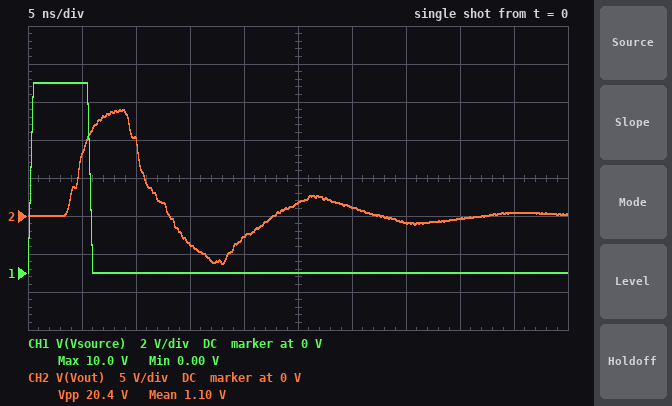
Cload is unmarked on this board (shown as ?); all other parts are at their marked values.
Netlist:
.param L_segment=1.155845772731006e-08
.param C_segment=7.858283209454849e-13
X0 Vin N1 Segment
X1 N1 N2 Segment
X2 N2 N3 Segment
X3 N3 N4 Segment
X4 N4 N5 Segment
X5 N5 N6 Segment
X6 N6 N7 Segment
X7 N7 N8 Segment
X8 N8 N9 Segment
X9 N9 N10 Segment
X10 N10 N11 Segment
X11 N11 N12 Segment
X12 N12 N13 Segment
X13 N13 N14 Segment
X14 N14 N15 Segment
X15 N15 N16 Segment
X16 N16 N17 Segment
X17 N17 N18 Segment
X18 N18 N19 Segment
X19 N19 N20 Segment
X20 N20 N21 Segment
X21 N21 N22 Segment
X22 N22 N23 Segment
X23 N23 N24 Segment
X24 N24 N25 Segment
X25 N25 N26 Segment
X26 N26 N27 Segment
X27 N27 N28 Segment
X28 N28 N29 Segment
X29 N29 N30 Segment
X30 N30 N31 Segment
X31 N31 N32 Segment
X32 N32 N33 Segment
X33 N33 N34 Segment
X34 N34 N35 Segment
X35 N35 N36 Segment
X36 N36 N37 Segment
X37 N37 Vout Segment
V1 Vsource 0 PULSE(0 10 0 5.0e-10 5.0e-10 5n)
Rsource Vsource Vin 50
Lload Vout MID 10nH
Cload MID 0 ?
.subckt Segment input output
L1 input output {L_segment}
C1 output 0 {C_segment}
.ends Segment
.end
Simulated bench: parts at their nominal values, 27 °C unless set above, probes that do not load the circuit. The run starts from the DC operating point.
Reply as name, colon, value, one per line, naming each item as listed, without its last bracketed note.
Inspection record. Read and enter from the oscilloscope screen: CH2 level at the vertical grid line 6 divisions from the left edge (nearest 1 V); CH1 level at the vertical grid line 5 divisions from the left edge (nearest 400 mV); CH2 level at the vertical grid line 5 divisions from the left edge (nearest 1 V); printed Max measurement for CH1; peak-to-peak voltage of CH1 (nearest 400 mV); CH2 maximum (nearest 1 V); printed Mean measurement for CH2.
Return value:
CH2 level at the vertical grid line 6 divisions from the left edge: 1 V
CH1 level at the vertical grid line 5 divisions from the left edge: 0 V
CH2 level at the vertical grid line 5 divisions from the left edge: 2 V
printed Max measurement for CH1: 10.0 V
peak-to-peak voltage of CH1: 10.0 V
CH2 maximum: 14 V
printed Mean measurement for CH2: 1.10 V
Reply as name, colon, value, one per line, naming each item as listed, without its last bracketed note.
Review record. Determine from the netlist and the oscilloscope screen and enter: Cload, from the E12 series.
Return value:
Cload, from the E12 series: 10 pF
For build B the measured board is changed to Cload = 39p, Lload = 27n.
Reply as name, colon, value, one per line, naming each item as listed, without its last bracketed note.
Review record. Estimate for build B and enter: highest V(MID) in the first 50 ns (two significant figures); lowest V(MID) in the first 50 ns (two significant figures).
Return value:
highest V(MID) in the first 50 ns: 9.7 V
lowest V(MID) in the first 50 ns: -2.9 V
